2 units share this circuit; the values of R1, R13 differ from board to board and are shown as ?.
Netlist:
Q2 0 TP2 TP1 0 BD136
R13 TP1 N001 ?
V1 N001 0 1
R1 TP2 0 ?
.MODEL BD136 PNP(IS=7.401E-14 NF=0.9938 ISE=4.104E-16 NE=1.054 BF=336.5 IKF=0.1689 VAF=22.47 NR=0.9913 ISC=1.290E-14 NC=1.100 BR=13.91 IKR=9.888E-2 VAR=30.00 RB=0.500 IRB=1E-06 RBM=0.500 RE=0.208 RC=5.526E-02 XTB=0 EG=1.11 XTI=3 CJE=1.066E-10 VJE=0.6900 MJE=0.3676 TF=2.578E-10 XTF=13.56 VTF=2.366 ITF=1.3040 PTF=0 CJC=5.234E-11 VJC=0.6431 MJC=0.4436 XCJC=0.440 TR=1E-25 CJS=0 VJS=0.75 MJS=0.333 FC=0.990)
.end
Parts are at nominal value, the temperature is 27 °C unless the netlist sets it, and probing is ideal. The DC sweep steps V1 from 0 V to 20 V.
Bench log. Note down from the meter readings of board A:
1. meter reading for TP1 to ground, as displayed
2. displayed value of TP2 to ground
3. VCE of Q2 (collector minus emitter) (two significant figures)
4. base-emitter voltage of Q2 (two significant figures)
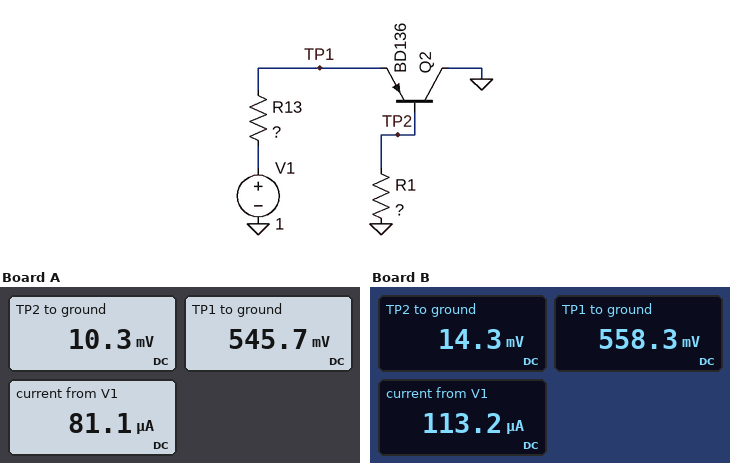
545.7 mV
10.3 mV
-550 mV
-540 mV
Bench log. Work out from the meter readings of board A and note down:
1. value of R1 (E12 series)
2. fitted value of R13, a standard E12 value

27 kΩ
5.6 kΩ
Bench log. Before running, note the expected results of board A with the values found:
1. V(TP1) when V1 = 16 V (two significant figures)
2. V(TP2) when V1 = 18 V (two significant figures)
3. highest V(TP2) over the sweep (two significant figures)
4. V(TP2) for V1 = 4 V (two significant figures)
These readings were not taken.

950 mV
360 mV
400 mV
73 mV
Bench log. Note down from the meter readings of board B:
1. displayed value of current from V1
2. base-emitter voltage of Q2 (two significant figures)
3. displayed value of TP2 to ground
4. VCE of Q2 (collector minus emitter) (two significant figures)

113.2 µA
-540 mV
14.3 mV
-560 mV
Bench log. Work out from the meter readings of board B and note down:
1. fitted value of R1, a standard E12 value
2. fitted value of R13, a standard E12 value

27 kΩ
3.9 kΩ
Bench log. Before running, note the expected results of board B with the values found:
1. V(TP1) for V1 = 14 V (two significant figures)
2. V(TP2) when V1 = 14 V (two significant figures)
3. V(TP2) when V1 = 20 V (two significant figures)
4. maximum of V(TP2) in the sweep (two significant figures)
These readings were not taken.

1.0 V
400 mV
570 mV
570 mV
